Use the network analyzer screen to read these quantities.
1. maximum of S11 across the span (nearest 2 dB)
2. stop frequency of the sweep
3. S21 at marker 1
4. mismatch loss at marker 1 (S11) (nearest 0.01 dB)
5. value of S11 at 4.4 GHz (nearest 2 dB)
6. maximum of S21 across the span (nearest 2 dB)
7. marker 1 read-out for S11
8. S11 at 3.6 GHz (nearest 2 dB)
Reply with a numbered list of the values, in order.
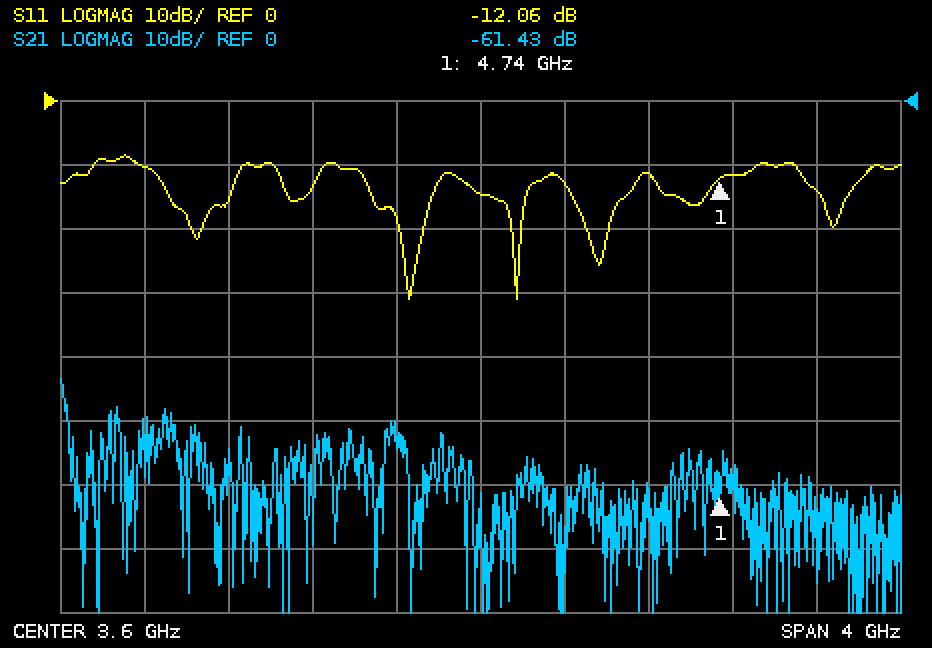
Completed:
1. -8 dB
2. 5.6 GHz
3. -61.43 dB
4. 0.28 dB
5. -12 dB
6. -44 dB
7. -12.06 dB
8. -14 dB
